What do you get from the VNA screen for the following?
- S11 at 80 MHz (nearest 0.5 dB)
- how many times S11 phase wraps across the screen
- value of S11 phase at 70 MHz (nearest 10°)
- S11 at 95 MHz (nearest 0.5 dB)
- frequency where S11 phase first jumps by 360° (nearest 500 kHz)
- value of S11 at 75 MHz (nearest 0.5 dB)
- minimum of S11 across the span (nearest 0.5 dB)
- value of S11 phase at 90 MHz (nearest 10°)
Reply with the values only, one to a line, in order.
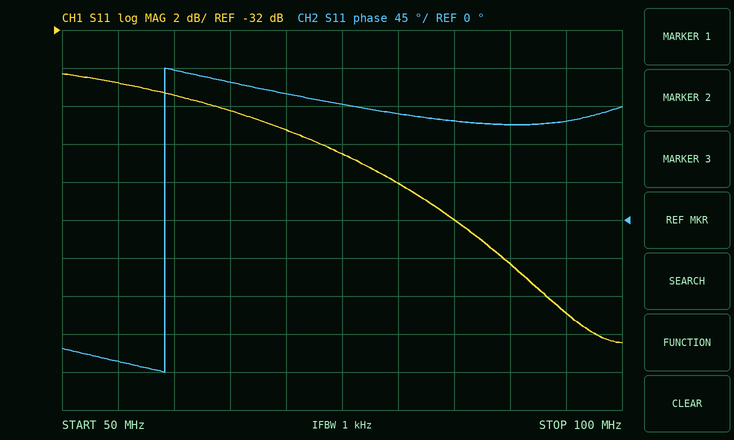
-40.0 dB
1
150°
-47.0 dB
59.0 MHz
-38.5 dB
-48.5 dB
110°
